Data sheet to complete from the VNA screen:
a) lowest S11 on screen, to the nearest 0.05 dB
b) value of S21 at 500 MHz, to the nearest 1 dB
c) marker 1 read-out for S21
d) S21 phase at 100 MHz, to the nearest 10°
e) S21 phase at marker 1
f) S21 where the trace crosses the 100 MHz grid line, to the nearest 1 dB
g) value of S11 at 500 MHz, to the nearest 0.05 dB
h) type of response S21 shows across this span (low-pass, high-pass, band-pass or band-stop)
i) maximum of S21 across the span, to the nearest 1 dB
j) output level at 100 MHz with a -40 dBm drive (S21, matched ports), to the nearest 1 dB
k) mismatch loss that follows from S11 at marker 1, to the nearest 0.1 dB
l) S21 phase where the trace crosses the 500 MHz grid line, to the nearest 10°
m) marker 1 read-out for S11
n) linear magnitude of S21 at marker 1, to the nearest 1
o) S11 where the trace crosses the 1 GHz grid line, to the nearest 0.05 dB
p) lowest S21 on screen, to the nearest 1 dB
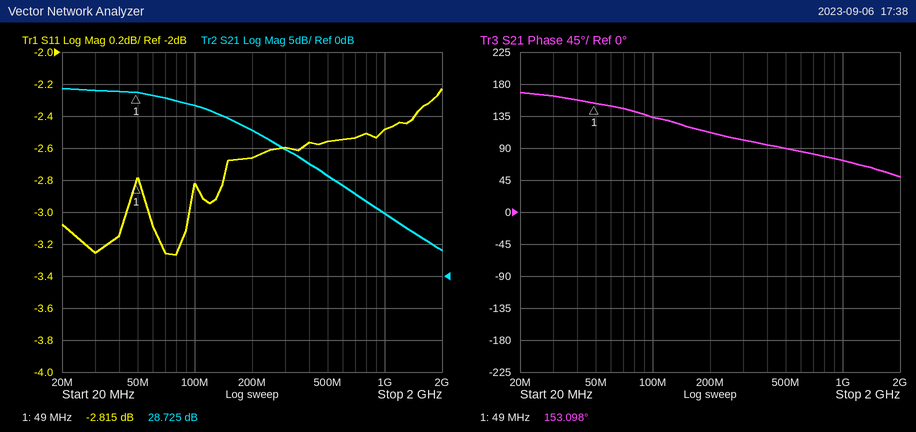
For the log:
-3.25 dB
16 dB
28.725 dB
130°
153.098°
27 dB
-2.55 dB
low-pass
29 dB
-13 dBm
3.2 dB
90°
-2.815 dB
27
-2.50 dB
4 dB
